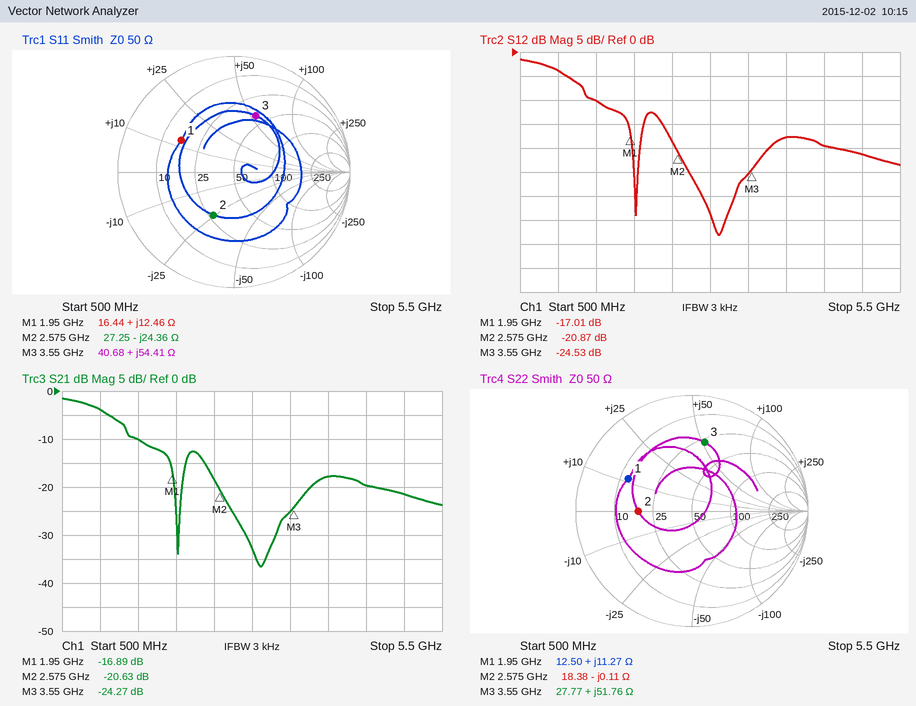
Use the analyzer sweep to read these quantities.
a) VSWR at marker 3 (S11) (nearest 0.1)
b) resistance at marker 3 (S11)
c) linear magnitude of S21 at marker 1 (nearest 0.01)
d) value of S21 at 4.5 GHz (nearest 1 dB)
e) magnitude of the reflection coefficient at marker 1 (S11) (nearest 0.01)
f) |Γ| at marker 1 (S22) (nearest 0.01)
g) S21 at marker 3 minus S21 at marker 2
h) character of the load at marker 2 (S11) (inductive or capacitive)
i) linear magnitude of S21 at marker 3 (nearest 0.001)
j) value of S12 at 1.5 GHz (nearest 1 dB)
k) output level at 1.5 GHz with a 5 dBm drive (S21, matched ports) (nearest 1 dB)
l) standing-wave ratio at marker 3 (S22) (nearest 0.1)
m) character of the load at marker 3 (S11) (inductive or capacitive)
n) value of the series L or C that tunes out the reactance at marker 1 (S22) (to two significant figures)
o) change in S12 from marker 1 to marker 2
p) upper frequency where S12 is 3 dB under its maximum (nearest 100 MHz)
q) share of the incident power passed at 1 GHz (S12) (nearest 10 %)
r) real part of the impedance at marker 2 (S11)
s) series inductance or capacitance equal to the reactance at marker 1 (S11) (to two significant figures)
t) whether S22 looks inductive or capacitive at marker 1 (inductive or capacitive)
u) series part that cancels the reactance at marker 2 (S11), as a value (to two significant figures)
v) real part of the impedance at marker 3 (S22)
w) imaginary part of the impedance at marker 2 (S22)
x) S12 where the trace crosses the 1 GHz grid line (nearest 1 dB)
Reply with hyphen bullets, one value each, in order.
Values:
- 3.2
- 40.68 Ω
- 0.14
- -20 dB
- 0.53
- 0.62
- -3.64 dB
- capacitive
- 0.061
- -10 dB
- -5 dBm
- 4.0
- inductive
- 7.2 pF
- -3.86 dB
- 1.1 GHz
- 40 %
- 27.25 Ω
- 1.0 nH
- inductive
- 1.5 nH
- 27.77 Ω
- -0.11 Ω
- -4 dB
